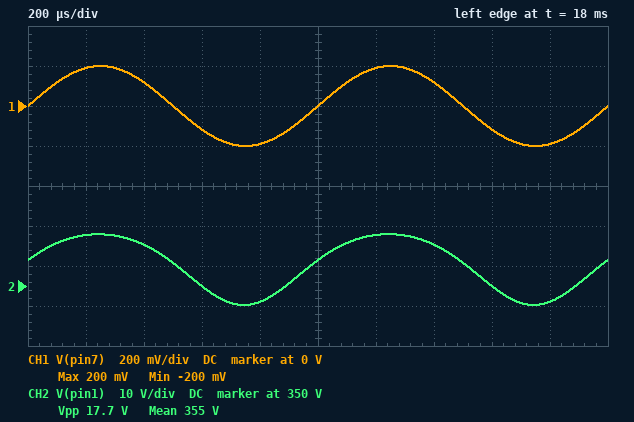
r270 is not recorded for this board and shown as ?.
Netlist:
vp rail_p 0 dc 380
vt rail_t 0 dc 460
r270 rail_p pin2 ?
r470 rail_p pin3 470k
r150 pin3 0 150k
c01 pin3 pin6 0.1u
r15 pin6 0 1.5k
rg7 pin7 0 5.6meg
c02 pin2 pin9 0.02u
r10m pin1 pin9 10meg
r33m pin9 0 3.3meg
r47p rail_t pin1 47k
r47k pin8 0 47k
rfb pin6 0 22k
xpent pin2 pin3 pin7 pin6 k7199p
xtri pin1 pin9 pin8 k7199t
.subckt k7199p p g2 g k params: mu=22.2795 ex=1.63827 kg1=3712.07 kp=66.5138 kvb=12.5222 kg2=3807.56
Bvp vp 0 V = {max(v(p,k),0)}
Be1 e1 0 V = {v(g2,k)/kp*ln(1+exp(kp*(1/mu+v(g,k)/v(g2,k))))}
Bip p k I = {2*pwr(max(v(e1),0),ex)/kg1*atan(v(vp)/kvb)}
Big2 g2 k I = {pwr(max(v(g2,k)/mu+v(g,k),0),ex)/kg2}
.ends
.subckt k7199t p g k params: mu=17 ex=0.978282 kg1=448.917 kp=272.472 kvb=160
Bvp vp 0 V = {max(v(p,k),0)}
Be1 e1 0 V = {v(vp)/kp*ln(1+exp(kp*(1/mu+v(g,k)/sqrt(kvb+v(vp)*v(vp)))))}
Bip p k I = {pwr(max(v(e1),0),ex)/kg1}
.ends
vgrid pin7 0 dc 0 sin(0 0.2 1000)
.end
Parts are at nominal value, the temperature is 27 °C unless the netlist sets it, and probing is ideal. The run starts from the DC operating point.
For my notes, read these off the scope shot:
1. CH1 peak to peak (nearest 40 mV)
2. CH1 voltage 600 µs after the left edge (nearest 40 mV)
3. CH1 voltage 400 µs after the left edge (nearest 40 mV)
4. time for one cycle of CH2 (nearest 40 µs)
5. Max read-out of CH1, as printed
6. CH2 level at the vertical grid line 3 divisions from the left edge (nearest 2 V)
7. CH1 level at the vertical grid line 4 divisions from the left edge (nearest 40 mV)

400 mV
-120 mV
120 mV
1.00 ms
200 mV
350 V
-200 mV
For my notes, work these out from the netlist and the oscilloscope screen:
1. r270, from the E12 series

390 kΩ
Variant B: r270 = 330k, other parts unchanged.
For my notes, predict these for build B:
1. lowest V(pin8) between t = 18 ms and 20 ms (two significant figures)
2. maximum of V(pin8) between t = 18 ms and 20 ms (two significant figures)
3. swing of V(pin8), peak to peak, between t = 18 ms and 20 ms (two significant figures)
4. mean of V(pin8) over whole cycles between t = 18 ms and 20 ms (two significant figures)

91 V
120 V
27 V
100 V
